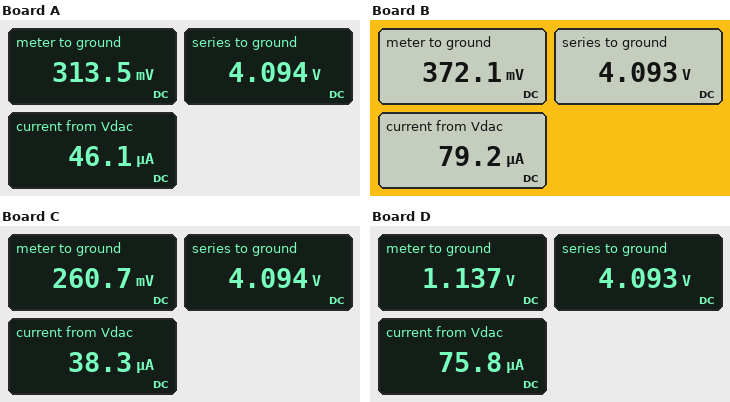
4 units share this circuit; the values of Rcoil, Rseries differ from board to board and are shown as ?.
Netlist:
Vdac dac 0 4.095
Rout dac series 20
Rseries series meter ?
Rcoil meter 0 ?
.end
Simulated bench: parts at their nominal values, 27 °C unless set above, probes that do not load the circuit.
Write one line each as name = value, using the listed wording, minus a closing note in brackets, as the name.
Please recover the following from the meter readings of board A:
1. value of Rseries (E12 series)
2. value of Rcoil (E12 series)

value of Rseries = 82 kΩ
value of Rcoil = 6.8 kΩ
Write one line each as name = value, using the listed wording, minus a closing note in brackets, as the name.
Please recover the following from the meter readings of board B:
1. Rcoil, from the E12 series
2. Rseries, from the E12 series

Rcoil, from the E12 series = 4.7 kΩ
Rseries, from the E12 series = 47 kΩ
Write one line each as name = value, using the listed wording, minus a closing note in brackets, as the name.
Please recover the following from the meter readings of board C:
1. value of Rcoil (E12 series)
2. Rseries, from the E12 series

value of Rcoil = 6.8 kΩ
Rseries, from the E12 series = 100 kΩ
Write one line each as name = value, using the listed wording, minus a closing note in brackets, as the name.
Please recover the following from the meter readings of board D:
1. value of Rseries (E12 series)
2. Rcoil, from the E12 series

value of Rseries = 39 kΩ
Rcoil, from the E12 series = 15 kΩ
